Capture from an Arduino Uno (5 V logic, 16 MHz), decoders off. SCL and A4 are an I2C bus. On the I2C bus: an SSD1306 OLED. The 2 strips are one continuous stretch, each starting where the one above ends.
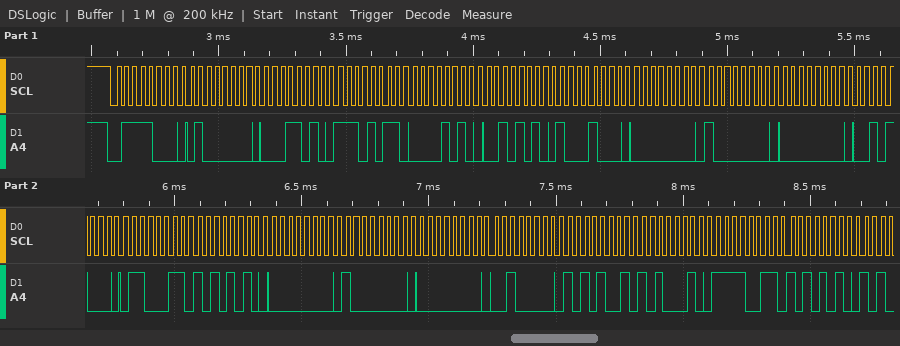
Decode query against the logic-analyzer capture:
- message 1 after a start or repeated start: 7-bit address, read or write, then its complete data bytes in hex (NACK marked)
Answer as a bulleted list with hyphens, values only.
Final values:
- 0x3C write: 40 1A EB 0A 2A 88 00 80 00 28 63 AA 00 80 00 20 A9 A2 F3 AA
